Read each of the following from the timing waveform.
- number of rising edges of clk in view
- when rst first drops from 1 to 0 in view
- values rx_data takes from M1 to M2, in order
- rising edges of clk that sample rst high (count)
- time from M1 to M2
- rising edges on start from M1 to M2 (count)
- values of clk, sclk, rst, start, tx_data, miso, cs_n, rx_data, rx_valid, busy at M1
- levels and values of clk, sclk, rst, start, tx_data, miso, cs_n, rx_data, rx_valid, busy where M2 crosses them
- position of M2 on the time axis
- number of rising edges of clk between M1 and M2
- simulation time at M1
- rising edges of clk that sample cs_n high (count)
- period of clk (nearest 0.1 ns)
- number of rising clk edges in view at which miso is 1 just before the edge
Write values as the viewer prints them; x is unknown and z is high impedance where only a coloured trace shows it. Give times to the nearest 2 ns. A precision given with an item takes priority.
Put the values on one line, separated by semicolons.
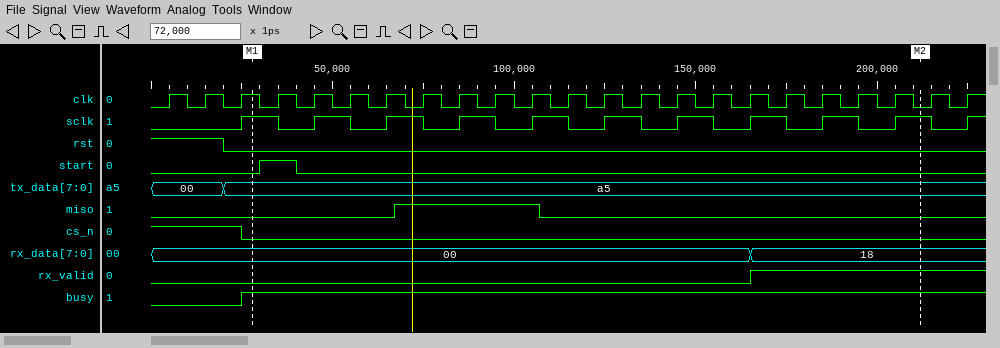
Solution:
23; 20 ns; 00, 18; 2; 184 ns; 1; clk=1, sclk=1, rst=0, start=0, tx_data=a5, miso=0, cs_n=0, rx_data=00, rx_valid=0, busy=1; clk=0, sclk=1, rst=0, start=0, tx_data=a5, miso=0, cs_n=0, rx_data=18, rx_valid=1, busy=1; 212 ns; 18; 28 ns; 3; 10 ns; 4
